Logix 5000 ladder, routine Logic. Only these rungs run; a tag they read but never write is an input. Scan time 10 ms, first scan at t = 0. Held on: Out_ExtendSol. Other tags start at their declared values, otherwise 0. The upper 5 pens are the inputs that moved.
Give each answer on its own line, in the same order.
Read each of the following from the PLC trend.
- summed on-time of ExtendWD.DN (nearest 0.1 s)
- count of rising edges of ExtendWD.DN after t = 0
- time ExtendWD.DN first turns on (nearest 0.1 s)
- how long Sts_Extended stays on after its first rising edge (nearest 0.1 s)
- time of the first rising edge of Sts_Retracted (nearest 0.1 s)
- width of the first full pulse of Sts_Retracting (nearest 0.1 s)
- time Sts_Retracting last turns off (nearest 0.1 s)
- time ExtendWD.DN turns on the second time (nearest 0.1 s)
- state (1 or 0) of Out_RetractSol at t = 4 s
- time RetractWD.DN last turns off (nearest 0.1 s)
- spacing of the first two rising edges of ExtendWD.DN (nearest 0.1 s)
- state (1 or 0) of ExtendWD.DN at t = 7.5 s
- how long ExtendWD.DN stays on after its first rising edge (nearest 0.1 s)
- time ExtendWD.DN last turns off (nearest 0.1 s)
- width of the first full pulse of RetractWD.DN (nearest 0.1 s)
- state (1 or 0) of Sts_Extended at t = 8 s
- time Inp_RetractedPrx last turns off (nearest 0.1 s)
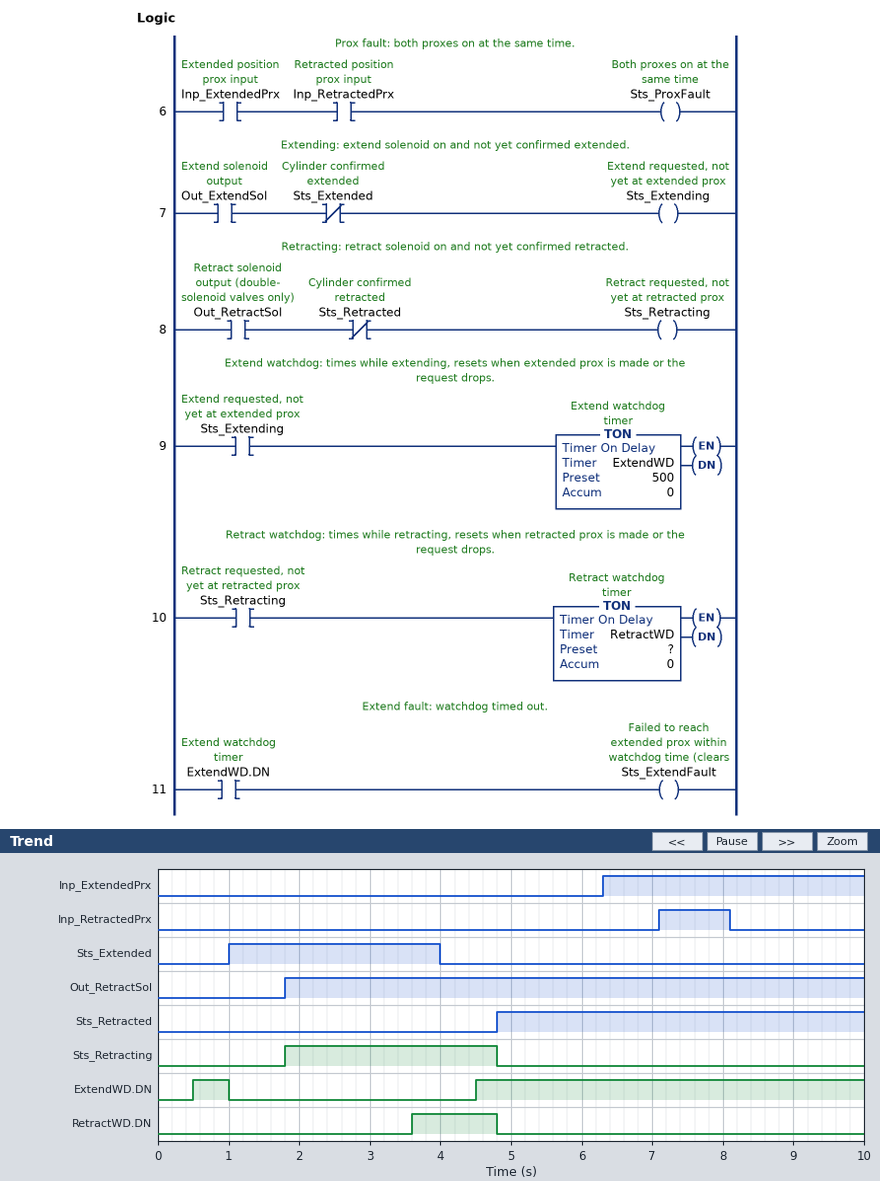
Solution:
6.0 s
2
0.5 s
3.0 s
4.8 s
3.0 s
4.8 s
4.5 s
1
4.8 s
4.0 s
1
0.5 s
1.0 s
1.2 s
0
8.1 s
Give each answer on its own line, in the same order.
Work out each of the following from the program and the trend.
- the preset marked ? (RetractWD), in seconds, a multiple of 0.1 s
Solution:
1.8 s
